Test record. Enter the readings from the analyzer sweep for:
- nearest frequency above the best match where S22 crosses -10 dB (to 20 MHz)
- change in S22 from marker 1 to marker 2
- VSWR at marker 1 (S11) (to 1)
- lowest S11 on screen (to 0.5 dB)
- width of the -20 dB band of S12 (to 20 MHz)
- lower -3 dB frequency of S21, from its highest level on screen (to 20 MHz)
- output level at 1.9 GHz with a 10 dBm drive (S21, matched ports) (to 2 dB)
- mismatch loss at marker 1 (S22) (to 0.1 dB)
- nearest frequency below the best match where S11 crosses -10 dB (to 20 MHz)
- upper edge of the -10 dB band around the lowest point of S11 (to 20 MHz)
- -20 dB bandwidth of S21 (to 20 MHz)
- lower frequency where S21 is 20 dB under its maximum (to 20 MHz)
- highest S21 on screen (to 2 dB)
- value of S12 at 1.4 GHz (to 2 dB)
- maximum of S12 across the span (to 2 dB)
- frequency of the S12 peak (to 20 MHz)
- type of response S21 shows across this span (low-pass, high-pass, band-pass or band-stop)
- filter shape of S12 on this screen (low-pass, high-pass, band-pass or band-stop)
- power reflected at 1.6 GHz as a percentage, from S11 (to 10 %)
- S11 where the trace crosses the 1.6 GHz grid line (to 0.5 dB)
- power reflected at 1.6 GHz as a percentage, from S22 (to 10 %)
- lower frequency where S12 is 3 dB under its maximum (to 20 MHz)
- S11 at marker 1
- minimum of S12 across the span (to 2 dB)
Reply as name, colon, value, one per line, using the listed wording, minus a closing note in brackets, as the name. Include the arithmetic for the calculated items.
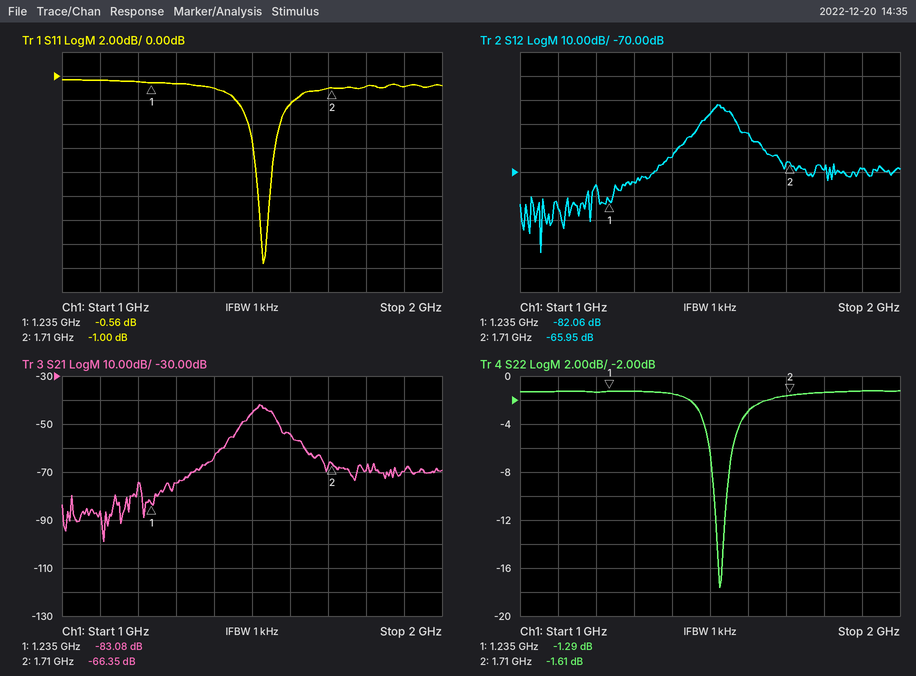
nearest frequency above the best match where S22 crosses -10 dB: 1.54 GHz
change in S22 from marker 1 to marker 2: -1.61 − (-1.29) = -0.32 dB
VSWR at marker 1 (S11): (1 + 0.9376)/(1 − 0.9376) ≈ 31
lowest S11 on screen: -15.5 dB
width of the -20 dB band of S12: 1.64 GHz − 1.40 GHz = 240 MHz
lower -3 dB frequency of S21, from its highest level on screen: 1.50 GHz
output level at 1.9 GHz with a 10 dBm drive (S21, matched ports): 10 dBm + (-70 dB) = -60 dBm
mismatch loss at marker 1 (S22): −10 log10(1 − 10^(-1.29/10)) ≈ 5.9 dB
nearest frequency below the best match where S11 crosses -10 dB: 1.52 GHz
upper edge of the -10 dB band around the lowest point of S11: 1.54 GHz
-20 dB bandwidth of S21: 1.64 GHz − 1.40 GHz = 240 MHz
lower frequency where S21 is 20 dB under its maximum: 1.40 GHz
highest S21 on screen: -42 dB
value of S12 at 1.4 GHz: -64 dB
maximum of S12 across the span: -42 dB
frequency of the S12 peak: 1.52 GHz
type of response S21 shows across this span: band-pass
filter shape of S12 on this screen: band-pass
power reflected at 1.6 GHz as a percentage, from S11: 10^(-2.5/10) ≈ 56.2 %, so 60 % to the nearest 10 %
S11 where the trace crosses the 1.6 GHz grid line: -2.5 dB
power reflected at 1.6 GHz as a percentage, from S22: 10^(-3/10) ≈ 50 %
lower frequency where S12 is 3 dB under its maximum: 1.50 GHz
S11 at marker 1: -0.56 dB
minimum of S12 across the span: -104 dB
